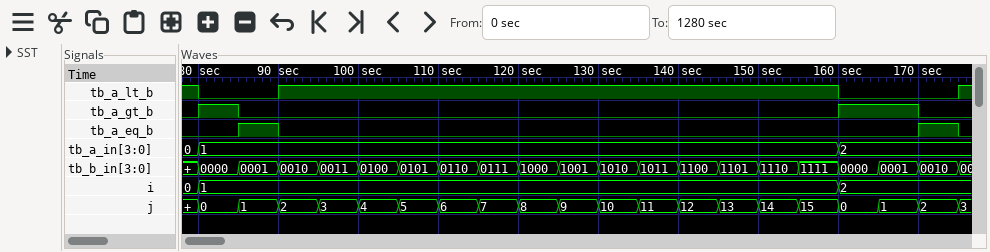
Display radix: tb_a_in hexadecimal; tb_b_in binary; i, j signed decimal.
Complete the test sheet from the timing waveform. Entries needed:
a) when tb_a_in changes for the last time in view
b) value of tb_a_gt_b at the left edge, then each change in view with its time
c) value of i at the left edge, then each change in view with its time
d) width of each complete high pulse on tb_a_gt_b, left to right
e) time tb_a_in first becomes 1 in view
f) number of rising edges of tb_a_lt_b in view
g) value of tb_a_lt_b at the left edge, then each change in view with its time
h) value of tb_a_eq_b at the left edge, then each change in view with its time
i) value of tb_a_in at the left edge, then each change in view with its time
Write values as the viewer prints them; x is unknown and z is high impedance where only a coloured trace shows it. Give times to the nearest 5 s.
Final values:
160 s
0, 1 at 80 s, 0 at 85 s, 1 at 160 s, 0 at 170 s
0, 1 at 80 s, 2 at 160 s
5 s, 10 s
80 s
2
1, 0 at 80 s, 1 at 90 s, 0 at 160 s, 1 at 175 s
0, 1 at 85 s, 0 at 90 s, 1 at 170 s, 0 at 175 s
0, 1 at 80 s, 2 at 160 s
